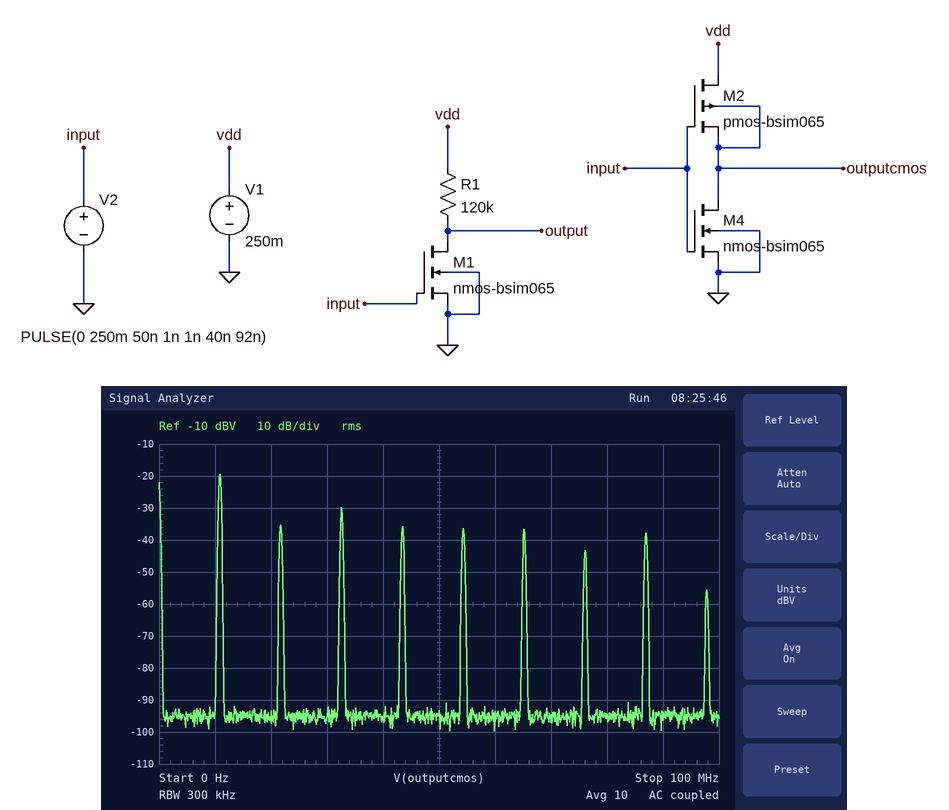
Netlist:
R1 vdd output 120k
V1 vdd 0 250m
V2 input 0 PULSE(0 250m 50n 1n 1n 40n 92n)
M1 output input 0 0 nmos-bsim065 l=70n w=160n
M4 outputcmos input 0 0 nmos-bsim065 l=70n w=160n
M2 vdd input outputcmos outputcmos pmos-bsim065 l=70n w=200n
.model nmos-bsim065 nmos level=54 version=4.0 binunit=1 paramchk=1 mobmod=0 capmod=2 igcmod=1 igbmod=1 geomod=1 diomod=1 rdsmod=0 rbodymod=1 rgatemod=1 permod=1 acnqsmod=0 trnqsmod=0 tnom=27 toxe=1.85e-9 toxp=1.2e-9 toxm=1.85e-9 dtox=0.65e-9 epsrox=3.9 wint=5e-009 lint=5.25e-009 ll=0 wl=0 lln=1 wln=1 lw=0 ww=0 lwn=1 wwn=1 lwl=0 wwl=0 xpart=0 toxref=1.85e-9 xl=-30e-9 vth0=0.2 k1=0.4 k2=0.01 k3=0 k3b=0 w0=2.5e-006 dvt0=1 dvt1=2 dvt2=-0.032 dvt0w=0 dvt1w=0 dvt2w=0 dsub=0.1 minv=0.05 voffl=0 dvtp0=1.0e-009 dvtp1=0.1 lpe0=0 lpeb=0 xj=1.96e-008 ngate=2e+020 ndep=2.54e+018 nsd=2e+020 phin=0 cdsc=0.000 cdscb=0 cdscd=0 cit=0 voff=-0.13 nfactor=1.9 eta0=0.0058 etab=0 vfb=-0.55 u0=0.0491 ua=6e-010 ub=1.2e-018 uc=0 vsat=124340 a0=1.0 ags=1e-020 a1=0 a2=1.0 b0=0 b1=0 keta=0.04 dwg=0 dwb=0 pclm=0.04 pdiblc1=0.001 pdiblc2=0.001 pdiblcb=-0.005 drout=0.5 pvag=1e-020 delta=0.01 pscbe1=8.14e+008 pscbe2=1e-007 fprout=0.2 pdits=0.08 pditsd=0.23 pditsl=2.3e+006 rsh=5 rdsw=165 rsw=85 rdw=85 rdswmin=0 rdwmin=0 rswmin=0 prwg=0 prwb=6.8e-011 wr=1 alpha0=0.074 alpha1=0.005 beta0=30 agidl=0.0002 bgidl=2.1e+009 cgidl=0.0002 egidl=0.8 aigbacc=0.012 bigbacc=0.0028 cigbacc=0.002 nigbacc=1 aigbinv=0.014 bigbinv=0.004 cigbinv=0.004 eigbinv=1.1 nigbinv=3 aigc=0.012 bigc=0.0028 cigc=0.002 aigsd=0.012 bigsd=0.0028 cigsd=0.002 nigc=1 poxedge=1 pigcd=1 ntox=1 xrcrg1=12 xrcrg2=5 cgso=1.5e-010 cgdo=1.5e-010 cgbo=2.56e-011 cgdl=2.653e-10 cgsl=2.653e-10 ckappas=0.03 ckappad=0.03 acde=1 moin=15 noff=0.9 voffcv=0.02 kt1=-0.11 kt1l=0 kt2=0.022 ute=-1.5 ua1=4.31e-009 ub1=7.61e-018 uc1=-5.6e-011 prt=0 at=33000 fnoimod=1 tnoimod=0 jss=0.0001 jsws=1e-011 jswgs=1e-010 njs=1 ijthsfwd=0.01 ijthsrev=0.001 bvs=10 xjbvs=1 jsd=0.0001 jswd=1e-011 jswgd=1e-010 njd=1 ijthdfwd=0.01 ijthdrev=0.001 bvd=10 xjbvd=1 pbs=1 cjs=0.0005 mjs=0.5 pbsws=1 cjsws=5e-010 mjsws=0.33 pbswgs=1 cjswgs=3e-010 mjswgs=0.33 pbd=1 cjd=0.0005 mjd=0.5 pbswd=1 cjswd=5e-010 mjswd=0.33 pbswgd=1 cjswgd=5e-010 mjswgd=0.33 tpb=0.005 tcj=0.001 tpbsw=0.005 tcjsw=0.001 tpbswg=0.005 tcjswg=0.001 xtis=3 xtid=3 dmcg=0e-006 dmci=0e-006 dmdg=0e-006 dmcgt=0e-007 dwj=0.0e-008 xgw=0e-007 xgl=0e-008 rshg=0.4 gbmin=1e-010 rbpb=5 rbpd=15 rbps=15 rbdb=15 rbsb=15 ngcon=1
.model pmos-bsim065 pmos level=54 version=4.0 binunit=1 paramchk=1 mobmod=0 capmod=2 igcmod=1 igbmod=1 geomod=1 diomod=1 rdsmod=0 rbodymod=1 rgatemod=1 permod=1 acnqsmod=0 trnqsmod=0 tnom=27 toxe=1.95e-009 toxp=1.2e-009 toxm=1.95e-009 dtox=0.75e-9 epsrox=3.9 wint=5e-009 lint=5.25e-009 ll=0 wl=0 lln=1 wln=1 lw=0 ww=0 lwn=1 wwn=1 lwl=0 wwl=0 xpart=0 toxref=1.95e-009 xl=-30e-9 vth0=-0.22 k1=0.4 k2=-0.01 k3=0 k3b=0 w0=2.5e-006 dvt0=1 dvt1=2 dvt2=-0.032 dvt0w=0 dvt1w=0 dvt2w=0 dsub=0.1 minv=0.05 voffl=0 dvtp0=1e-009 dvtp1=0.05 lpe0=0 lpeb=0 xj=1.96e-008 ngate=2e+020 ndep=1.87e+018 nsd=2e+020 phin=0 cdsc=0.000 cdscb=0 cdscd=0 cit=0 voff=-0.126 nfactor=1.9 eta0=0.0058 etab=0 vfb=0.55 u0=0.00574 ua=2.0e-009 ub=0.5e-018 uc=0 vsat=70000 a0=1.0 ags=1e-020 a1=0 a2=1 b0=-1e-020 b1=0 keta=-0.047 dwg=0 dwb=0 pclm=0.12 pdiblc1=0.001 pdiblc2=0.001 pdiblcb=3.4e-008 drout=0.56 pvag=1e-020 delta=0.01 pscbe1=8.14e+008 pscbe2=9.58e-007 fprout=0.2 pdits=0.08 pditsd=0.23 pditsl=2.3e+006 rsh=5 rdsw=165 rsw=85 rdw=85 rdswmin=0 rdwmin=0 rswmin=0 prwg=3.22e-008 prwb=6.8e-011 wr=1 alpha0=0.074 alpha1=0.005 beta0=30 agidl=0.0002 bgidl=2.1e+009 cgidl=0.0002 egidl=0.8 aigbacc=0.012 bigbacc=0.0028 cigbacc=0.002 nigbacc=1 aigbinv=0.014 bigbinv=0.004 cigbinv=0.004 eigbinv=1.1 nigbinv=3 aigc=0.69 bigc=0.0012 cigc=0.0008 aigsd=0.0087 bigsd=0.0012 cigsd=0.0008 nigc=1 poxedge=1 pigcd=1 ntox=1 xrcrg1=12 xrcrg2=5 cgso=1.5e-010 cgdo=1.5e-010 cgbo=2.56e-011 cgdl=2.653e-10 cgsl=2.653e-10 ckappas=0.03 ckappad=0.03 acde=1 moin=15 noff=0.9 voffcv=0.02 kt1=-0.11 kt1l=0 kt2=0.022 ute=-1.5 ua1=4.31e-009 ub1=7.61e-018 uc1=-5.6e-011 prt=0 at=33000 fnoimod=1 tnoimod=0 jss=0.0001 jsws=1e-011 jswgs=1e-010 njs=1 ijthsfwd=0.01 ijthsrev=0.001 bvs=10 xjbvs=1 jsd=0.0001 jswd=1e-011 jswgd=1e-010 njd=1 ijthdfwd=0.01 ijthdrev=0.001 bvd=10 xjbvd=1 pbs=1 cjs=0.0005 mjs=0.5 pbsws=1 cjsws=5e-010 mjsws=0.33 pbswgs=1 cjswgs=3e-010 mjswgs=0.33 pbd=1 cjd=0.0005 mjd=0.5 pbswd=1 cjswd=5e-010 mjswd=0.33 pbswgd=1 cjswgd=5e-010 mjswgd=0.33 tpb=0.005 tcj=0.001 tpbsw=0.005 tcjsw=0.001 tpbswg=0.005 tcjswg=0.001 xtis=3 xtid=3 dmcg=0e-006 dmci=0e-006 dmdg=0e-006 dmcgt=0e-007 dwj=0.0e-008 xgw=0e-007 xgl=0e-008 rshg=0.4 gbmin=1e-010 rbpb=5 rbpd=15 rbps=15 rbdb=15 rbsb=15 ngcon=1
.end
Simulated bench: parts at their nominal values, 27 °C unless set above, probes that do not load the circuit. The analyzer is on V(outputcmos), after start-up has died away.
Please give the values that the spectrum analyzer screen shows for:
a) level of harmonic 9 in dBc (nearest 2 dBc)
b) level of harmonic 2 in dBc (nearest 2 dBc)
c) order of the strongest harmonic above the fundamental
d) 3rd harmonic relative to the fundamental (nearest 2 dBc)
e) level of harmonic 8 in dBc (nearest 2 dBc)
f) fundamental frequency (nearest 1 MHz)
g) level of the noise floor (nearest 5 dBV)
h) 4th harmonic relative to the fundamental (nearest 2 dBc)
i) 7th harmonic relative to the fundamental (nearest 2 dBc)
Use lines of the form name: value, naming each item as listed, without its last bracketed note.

level of harmonic 9 in dBc: -36 dBc
level of harmonic 2 in dBc: -16 dBc
order of the strongest harmonic above the fundamental: 3
3rd harmonic relative to the fundamental: -10 dBc
level of harmonic 8 in dBc: -18 dBc
fundamental frequency: 11 MHz
level of the noise floor: -95 dBV
4th harmonic relative to the fundamental: -16 dBc
7th harmonic relative to the fundamental: -24 dBc
